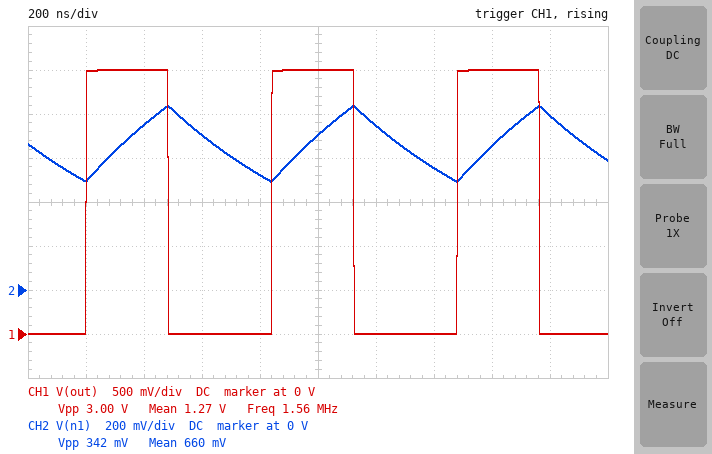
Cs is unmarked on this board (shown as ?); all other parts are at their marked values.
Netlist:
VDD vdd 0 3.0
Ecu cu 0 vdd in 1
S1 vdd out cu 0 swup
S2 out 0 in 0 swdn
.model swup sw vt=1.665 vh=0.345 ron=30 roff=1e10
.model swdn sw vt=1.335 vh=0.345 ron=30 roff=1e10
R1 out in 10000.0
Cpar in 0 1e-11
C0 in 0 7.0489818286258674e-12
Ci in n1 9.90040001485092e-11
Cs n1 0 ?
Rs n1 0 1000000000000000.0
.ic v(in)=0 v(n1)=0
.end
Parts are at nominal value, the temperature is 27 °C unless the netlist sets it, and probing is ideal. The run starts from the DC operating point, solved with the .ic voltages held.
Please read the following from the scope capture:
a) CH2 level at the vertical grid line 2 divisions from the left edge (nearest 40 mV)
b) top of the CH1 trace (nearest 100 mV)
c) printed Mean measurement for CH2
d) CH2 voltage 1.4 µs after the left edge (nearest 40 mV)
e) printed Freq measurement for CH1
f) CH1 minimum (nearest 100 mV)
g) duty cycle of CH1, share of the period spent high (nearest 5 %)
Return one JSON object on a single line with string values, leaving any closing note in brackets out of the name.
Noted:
{"CH2 level at the vertical grid line 2 divisions from the left edge": "760 mV", "top of the CH1 trace": "3.0 V", "printed Mean measurement for CH2": "660 mV", "CH2 voltage 1.4 µs after the left edge": "560 mV", "printed Freq measurement for CH1": "1.56 MHz", "CH1 minimum": "0 V", "duty cycle of CH1, share of the period spent high": "45 %"}
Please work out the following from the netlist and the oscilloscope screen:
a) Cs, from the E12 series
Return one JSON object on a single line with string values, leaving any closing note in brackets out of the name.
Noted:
{"Cs, from the E12 series": "100 pF"}
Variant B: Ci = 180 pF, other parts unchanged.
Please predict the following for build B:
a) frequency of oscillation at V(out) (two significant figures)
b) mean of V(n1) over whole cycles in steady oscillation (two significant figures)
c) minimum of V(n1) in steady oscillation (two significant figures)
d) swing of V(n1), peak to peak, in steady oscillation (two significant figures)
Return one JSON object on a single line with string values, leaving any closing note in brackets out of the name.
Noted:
{"frequency of oscillation at V(out)": "1.3 MHz", "mean of V(n1) over whole cycles in steady oscillation": "850 mV", "minimum of V(n1) in steady oscillation": "640 mV", "swing of V(n1), peak to peak, in steady oscillation": "440 mV"}
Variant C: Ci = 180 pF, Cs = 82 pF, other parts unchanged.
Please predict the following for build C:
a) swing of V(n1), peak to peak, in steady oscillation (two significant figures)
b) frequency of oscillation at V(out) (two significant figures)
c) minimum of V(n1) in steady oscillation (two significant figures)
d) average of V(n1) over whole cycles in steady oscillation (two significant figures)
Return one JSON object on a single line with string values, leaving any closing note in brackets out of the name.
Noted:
{"swing of V(n1), peak to peak, in steady oscillation": "470 mV", "frequency of oscillation at V(out)": "1.4 MHz", "minimum of V(n1) in steady oscillation": "680 mV", "average of V(n1) over whole cycles in steady oscillation": "910 mV"}
